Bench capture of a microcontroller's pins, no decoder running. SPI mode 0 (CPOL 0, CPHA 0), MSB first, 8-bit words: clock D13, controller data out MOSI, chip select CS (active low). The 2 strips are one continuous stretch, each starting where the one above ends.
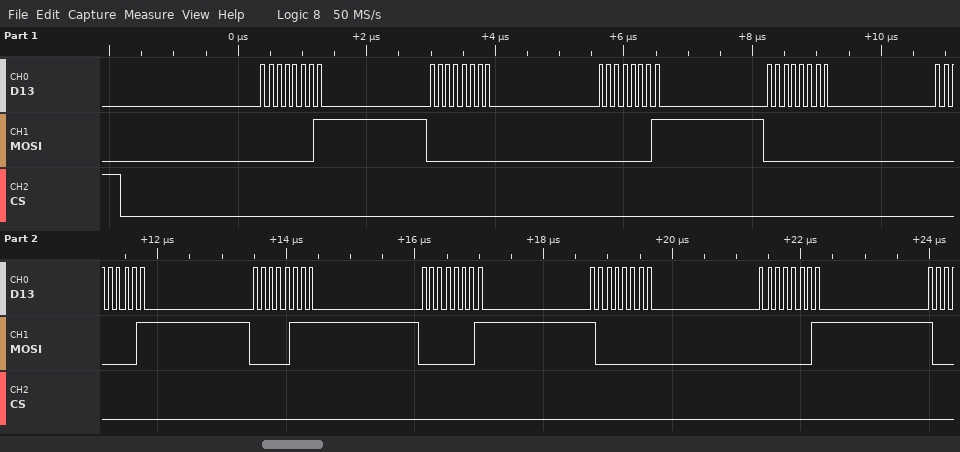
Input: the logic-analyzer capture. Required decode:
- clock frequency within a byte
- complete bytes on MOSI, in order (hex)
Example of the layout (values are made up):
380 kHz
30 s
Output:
8 MHz
0x01 0x00 0x01 0x00 0x01 0x07 0x01 0x80 0x01
